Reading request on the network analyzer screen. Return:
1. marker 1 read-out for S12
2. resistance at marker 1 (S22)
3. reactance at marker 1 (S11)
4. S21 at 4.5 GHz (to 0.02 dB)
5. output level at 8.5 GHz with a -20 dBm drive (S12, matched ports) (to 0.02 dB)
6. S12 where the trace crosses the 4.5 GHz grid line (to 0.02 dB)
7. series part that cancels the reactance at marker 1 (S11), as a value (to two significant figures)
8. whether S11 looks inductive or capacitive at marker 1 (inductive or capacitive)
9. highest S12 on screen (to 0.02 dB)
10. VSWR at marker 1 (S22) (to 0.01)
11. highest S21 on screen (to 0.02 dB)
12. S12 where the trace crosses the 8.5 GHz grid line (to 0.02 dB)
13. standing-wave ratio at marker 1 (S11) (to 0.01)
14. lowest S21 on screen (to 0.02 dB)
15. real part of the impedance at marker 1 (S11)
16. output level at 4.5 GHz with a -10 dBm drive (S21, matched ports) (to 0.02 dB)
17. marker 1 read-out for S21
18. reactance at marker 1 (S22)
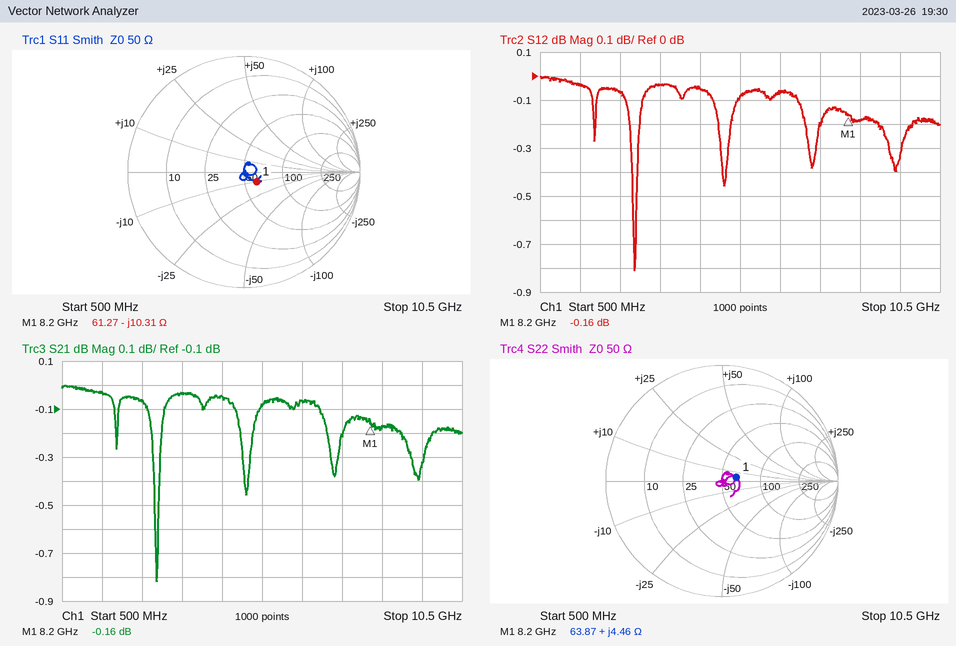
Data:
-0.16 dB
63.87 Ω
-10.31 Ω
-0.04 dB
-20.18 dBm
-0.06 dB
200 pH
capacitive
0.00 dB
1.29
0.00 dB
-0.18 dB
1.32
-0.82 dB
61.27 Ω
-10.04 dBm
-0.16 dB
+4.46 Ω
